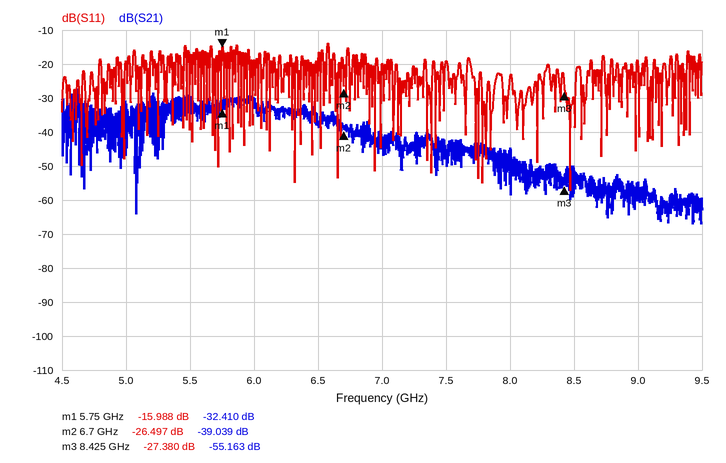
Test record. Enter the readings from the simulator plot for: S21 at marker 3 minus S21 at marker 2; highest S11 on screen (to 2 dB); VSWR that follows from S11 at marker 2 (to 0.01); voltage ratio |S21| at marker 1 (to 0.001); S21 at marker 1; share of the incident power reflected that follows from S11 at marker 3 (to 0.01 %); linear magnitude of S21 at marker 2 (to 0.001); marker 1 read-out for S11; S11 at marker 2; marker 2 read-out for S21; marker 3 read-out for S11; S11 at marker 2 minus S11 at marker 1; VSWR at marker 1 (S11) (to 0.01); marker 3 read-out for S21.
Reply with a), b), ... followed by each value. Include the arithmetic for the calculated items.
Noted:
a) -55.163 − (-39.039) = -16.124 dB
b) -14 dB
c) (1 + 0.0473)/(1 − 0.0473) ≈ 1.10
d) 10^(-32.41/20) ≈ 0.024
e) -32.410 dB
f) 10^(-27.38/10) ≈ 0.18 %
g) 10^(-39.039/20) ≈ 0.011
h) -15.988 dB
i) -26.497 dB
j) -39.039 dB
k) -27.380 dB
l) -26.497 − (-15.988) = -10.509 dB
m) (1 + 0.1587)/(1 − 0.1587) ≈ 1.38
n) -55.163 dB
